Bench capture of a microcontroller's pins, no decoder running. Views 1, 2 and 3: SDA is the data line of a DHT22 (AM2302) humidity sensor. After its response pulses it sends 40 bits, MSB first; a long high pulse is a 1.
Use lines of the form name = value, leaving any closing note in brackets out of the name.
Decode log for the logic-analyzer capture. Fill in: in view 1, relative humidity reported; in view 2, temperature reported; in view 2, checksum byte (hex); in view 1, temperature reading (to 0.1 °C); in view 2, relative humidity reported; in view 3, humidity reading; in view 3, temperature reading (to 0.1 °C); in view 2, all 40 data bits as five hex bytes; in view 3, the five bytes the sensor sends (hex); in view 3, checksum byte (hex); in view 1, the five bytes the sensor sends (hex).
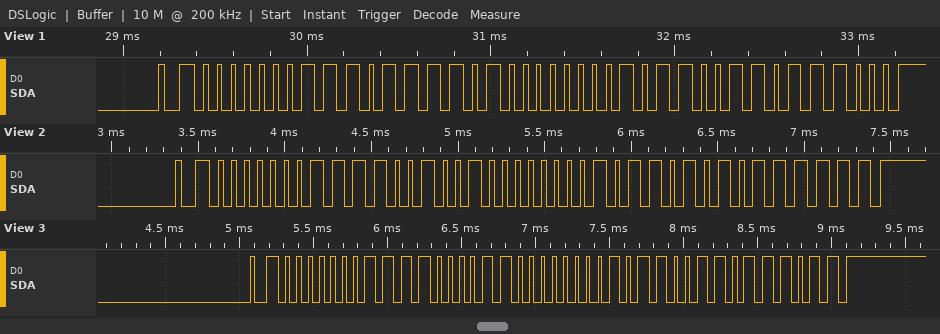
in view 1, relative humidity reported = 47.8 %
in view 2, temperature reported = -9.0 °C
in view 2, checksum byte = 0xBF
in view 1, temperature reading = -8.9 °C
in view 2, relative humidity reported = 48.4 %
in view 3, humidity reading = 48.1 %
in view 3, temperature reading = -8.9 °C
in view 2, all 40 data bits as five hex bytes = 01 E4 80 5A BF
in view 3, the five bytes the sensor sends = 01 E1 80 59 BB
in view 3, checksum byte = 0xBB
in view 1, the five bytes the sensor sends = 01 DE 80 59 B8
